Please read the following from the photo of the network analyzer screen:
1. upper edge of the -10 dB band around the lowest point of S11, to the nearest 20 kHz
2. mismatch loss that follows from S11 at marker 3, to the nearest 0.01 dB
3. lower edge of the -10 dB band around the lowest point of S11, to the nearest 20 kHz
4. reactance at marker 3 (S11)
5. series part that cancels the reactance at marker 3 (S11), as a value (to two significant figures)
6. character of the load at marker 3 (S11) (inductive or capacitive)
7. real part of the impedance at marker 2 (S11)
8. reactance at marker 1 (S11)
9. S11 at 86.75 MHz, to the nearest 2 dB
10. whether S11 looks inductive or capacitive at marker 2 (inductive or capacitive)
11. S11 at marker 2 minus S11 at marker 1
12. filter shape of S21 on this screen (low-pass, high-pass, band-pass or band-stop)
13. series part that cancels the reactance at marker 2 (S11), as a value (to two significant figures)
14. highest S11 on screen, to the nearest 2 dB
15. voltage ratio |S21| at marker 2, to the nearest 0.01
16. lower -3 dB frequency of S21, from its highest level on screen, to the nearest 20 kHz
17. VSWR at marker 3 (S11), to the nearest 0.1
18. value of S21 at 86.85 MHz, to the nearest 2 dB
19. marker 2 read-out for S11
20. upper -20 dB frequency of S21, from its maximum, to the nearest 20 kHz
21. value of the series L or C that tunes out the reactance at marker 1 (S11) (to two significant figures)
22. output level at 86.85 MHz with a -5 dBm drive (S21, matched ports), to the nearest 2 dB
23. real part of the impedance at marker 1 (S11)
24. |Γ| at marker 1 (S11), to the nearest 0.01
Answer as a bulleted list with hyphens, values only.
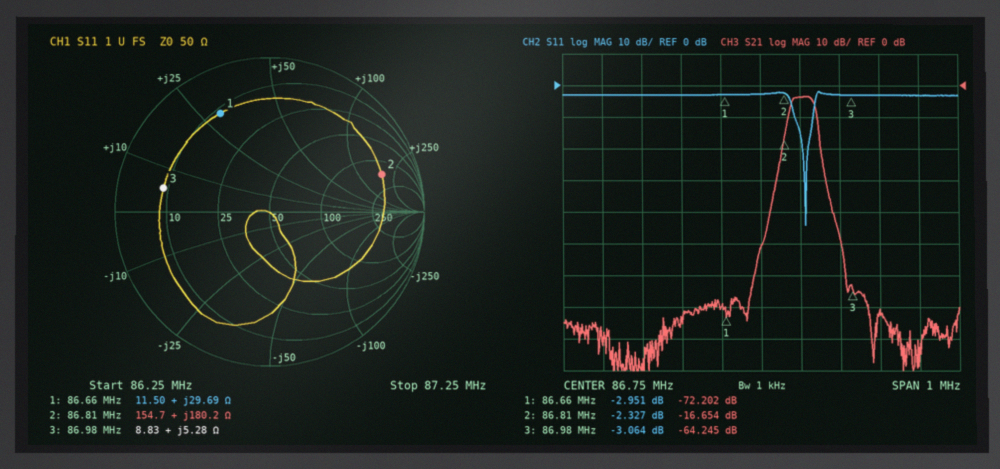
- 86.88 MHz
- 2.96 dB
- 86.84 MHz
- +5.28 Ω
- 350 pF
- inductive
- 154.7 Ω
- +29.69 Ω
- -2 dB
- inductive
- 0.624 dB
- band-pass
- 10 pF
- -2 dB
- 0.15
- 86.82 MHz
- 5.7
- -4 dB
- -2.327 dB
- 86.90 MHz
- 62 pF
- -8 dBm
- 11.50 Ω
- 0.71
